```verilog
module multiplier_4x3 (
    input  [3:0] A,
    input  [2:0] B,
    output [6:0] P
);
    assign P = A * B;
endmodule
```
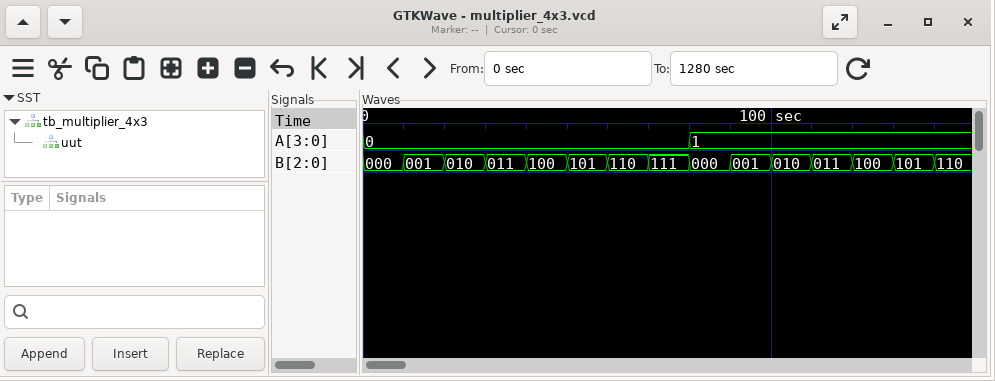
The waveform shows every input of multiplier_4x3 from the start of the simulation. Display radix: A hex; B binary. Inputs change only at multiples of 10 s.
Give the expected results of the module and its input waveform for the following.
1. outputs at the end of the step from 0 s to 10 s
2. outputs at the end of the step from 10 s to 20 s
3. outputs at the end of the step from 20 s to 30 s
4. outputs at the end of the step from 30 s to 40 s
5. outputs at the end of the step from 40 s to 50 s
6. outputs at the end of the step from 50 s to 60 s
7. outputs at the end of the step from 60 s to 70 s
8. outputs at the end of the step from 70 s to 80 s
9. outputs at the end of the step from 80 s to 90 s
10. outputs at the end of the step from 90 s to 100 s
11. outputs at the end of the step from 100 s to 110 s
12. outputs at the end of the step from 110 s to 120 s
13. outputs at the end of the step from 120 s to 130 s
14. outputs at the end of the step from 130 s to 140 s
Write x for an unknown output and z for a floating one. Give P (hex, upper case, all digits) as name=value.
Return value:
P=00
P=00
P=00
P=00
P=00
P=00
P=00
P=00
P=00
P=01
P=02
P=03
P=04
P=05
